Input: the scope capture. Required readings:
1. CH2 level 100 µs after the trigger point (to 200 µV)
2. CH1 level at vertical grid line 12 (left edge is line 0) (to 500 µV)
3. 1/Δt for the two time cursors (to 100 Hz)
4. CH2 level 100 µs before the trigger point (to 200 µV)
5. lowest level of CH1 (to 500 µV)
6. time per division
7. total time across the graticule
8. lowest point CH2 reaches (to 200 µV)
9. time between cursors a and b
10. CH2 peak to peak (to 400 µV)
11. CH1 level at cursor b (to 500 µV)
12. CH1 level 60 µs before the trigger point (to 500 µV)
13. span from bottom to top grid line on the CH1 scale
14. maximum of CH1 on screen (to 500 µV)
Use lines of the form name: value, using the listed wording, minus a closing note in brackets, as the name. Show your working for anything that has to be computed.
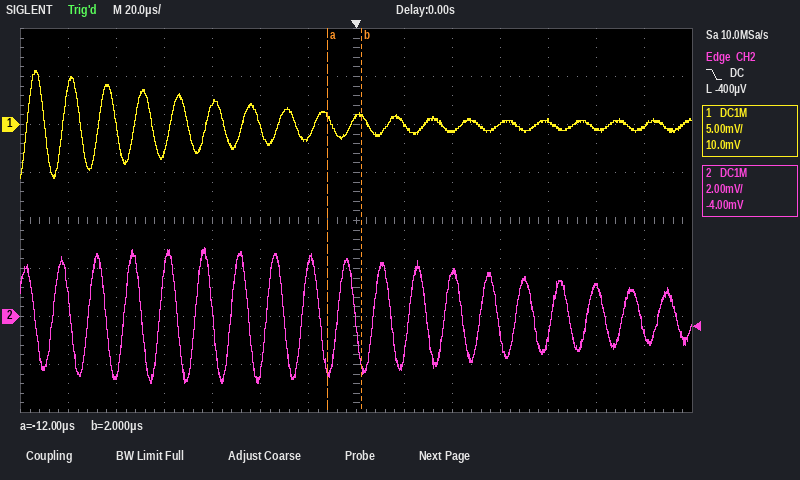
CH2 level 100 µs after the trigger point: 1.2 mV
CH1 level at vertical grid line 12 (left edge is line 0): -500 µV
1/Δt for the two time cursors: 1 / 14 µs ≈ 71.4 kHz
CH2 level 100 µs before the trigger point: -2.4 mV
lowest level of CH1: -5.5 mV
time per division: 20 µs
total time across the graticule: 280 µs
lowest point CH2 reaches: -2.8 mV
time between cursors a and b: 2 µs − (-12 µs) = 14 µs
CH2 peak to peak: 5.6 mV
CH1 level at cursor b: 1.0 mV
CH1 level 60 µs before the trigger point: 2.0 mV
span from bottom to top grid line on the CH1 scale: 40 mV
maximum of CH1 on screen: 5.5 mV
